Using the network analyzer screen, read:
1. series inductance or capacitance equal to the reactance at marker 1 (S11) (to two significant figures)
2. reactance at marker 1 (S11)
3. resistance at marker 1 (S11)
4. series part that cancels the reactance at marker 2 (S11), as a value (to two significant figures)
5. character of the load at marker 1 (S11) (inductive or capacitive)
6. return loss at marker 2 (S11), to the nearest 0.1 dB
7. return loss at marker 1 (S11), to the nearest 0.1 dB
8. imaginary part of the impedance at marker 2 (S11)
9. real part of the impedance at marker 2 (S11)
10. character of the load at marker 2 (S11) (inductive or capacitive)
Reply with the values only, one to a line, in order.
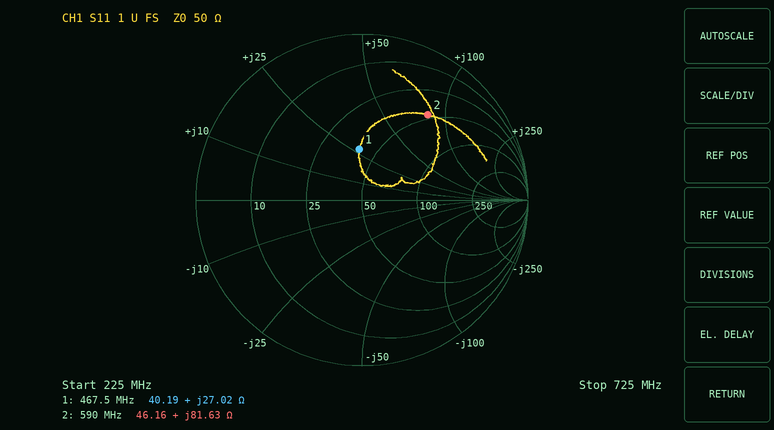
9.2 nH
+27.02 Ω
40.19 Ω
3.3 pF
inductive
3.8 dB
10.3 dB
+81.63 Ω
46.16 Ω
inductive
